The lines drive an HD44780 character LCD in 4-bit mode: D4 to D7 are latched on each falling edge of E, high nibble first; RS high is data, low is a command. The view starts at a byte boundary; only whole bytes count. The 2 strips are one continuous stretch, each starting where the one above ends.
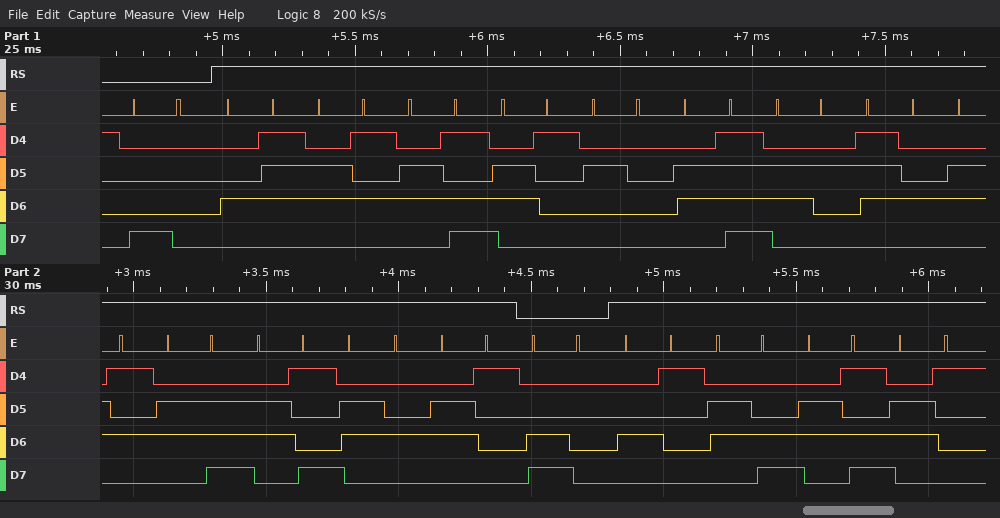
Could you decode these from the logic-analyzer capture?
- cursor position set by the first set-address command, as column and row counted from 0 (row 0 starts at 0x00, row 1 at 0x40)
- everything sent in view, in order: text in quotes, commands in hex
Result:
column 0, row 0
0x80 "Gema obtenida" 0xC0 "Alma"
